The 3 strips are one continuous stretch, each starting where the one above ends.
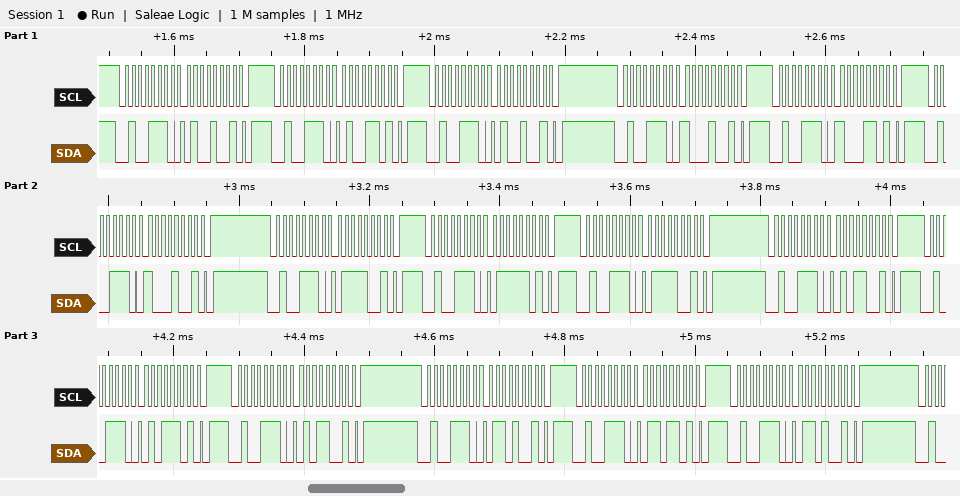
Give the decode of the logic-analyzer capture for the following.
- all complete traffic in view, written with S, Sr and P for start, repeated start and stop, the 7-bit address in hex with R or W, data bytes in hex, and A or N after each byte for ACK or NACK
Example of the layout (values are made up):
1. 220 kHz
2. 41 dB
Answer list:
1. S 27W A 49 A P S 27W A 4D A P S 27W A 49 A P S 27W A 89 A P S 27W A 8D A P S 27W A 89 A P S 27W A 79 A P S 27W A 7D A P S 27W A 79 A P S 27W A 59 A P S 27W A 5D A P S 27W A 59 A P S 27W A 69 A P S 27W A 6D A P S 27W A 69 A P
